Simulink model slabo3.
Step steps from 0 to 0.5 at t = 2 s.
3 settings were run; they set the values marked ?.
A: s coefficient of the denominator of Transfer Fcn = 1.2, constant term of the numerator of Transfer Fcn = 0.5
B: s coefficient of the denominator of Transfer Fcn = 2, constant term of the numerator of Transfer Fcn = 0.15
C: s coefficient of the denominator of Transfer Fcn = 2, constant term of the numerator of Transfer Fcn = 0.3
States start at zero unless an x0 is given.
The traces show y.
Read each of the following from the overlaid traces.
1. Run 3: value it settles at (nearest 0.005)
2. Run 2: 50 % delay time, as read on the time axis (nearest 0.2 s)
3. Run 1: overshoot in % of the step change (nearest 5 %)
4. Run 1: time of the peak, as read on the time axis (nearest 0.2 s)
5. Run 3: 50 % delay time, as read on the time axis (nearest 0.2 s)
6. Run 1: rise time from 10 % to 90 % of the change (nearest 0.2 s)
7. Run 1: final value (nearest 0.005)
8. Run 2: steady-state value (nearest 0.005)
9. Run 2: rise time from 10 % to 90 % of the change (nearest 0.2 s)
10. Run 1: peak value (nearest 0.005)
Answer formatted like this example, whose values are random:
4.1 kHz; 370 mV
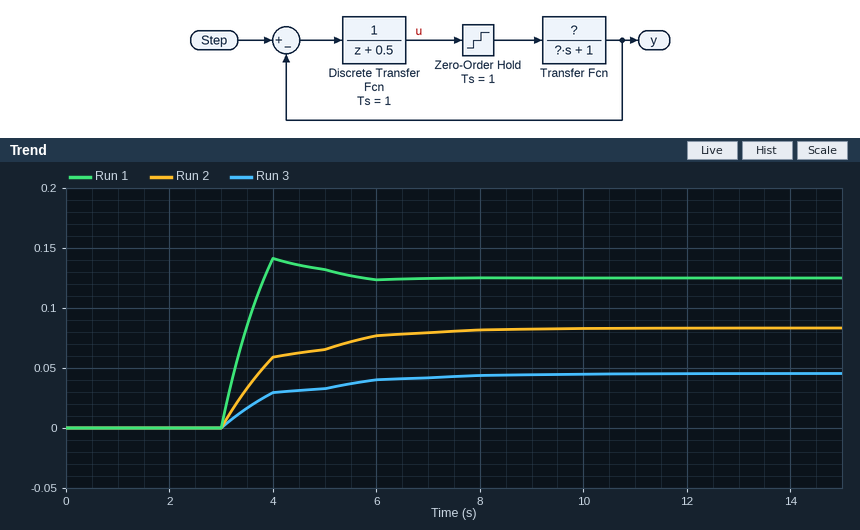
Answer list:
0.045; 3.6 s; 15 %; 4.0 s; 3.8 s; 0.6 s; 0.125; 0.085; 2.6 s; 0.140
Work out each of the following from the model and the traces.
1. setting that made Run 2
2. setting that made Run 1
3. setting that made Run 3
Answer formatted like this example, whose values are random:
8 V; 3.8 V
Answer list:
C; A; B
